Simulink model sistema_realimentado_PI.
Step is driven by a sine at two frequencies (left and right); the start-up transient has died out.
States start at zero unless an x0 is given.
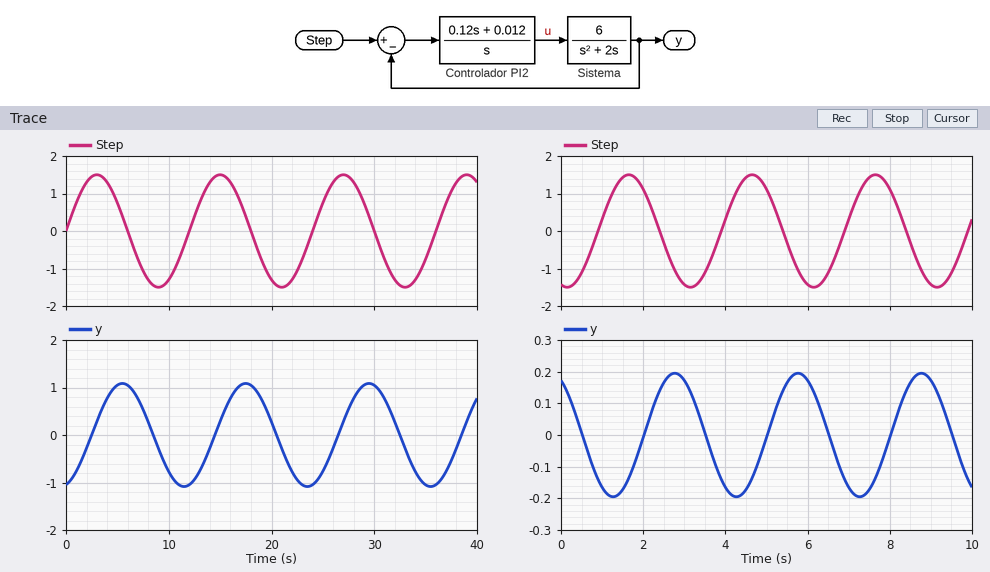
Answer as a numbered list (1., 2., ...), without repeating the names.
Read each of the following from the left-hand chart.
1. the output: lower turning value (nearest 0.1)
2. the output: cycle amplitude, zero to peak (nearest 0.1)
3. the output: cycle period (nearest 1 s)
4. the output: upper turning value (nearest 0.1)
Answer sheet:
1. -1.1
2. 1.1
3. 12 s
4. 1.1
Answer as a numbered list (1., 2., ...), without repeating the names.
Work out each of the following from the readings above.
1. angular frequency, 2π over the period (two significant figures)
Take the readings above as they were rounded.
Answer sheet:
1. 0.52 rad/s
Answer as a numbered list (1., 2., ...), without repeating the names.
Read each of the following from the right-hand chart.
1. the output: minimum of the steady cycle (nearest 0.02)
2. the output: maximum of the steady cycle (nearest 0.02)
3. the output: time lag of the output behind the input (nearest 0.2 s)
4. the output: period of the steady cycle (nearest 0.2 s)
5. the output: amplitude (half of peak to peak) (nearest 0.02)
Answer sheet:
1. -0.20
2. 0.20
3. 1.2 s
4. 3.0 s
5. 0.20
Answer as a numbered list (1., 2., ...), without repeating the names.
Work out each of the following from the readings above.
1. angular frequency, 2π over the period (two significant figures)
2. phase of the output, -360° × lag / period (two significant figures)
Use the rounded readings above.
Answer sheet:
1. 2.1 rad/s
2. -140°
